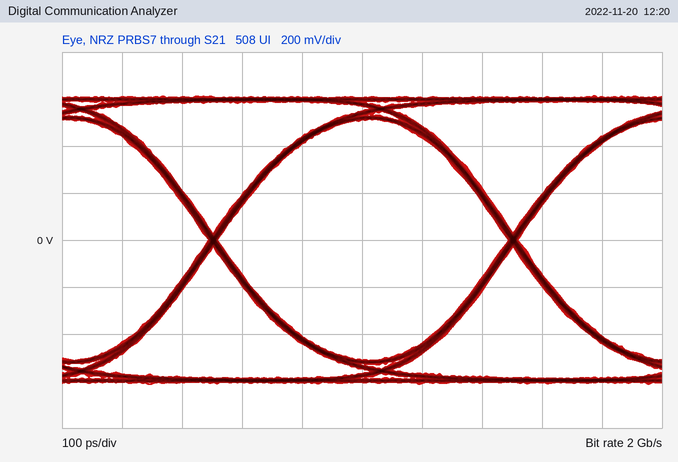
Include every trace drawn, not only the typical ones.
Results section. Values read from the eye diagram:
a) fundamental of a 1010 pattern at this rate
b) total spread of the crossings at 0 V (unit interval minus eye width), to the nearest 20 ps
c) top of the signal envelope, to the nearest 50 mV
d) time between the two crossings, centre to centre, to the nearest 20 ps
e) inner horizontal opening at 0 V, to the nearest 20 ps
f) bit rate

1 GHz
20 ps
600 mV
500 ps
480 ps
2 Gb/s
